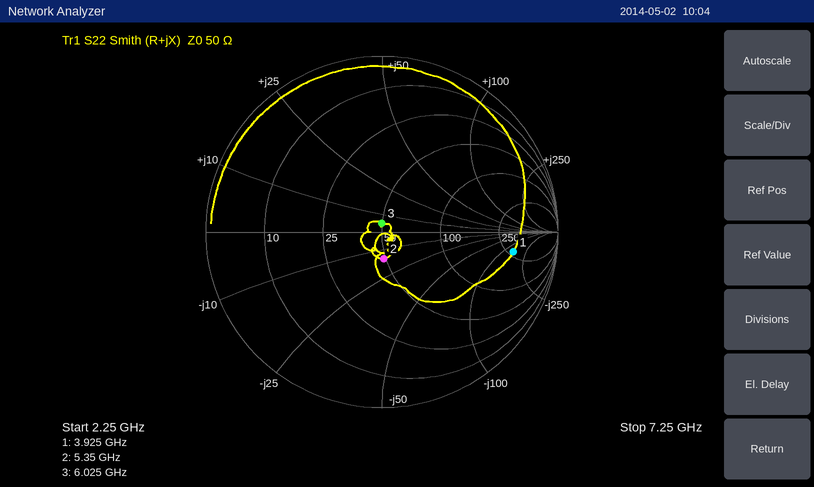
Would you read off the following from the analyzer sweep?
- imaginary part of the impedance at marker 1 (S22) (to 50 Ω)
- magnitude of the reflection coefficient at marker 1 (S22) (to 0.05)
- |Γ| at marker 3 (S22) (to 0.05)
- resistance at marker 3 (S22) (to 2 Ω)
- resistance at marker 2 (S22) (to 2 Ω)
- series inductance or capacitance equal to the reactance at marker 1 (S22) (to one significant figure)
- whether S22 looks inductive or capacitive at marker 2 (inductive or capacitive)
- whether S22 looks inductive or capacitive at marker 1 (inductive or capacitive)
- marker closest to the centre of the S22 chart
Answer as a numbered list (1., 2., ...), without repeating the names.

1. -150 Ω
2. 0.75
3. 0.05
4. 50 Ω
5. 48 Ω
6. 300 fF
7. capacitive
8. capacitive
9. marker 3
